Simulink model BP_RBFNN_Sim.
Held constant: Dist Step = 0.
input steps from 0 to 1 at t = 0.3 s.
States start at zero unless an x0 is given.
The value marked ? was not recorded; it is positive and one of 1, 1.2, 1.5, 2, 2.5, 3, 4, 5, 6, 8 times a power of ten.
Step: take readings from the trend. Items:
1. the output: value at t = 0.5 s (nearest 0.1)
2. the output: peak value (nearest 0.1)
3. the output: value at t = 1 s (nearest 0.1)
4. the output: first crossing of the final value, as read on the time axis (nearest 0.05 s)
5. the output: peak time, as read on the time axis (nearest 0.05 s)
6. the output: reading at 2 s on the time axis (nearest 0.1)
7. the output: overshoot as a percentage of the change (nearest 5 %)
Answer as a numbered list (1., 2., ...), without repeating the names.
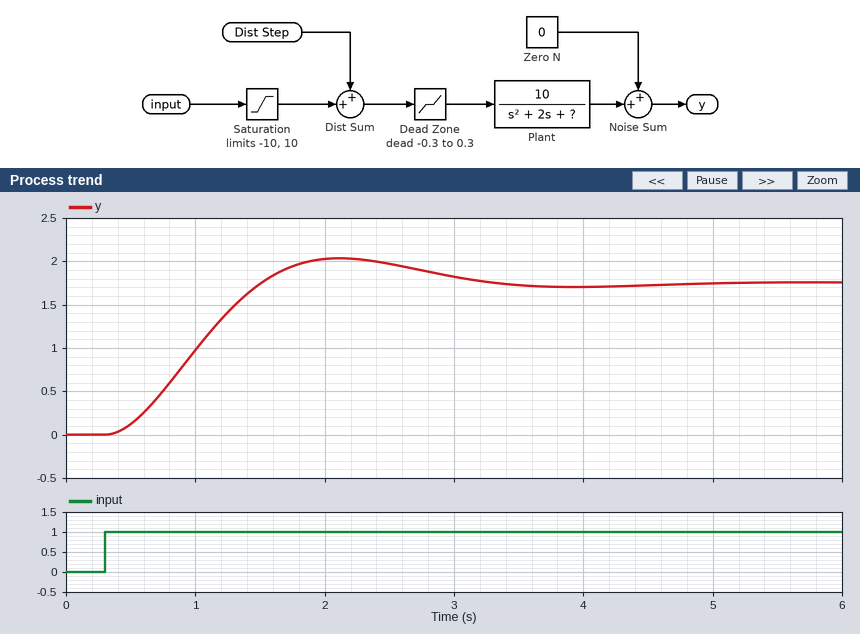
1. 0.1
2. 2.0
3. 1.0
4. 1.50 s
5. 2.10 s
6. 2.0
7. 15 %
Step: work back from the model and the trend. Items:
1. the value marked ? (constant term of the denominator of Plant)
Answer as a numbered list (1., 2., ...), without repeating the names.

1. 4
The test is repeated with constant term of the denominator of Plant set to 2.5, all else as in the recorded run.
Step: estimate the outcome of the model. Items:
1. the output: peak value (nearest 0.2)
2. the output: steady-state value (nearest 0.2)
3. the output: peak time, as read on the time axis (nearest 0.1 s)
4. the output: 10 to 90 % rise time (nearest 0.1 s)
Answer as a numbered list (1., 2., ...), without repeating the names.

1. 3.0
2. 2.8
3. 2.9 s
4. 1.2 s
